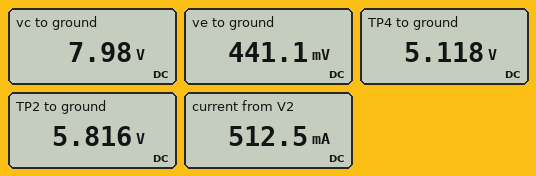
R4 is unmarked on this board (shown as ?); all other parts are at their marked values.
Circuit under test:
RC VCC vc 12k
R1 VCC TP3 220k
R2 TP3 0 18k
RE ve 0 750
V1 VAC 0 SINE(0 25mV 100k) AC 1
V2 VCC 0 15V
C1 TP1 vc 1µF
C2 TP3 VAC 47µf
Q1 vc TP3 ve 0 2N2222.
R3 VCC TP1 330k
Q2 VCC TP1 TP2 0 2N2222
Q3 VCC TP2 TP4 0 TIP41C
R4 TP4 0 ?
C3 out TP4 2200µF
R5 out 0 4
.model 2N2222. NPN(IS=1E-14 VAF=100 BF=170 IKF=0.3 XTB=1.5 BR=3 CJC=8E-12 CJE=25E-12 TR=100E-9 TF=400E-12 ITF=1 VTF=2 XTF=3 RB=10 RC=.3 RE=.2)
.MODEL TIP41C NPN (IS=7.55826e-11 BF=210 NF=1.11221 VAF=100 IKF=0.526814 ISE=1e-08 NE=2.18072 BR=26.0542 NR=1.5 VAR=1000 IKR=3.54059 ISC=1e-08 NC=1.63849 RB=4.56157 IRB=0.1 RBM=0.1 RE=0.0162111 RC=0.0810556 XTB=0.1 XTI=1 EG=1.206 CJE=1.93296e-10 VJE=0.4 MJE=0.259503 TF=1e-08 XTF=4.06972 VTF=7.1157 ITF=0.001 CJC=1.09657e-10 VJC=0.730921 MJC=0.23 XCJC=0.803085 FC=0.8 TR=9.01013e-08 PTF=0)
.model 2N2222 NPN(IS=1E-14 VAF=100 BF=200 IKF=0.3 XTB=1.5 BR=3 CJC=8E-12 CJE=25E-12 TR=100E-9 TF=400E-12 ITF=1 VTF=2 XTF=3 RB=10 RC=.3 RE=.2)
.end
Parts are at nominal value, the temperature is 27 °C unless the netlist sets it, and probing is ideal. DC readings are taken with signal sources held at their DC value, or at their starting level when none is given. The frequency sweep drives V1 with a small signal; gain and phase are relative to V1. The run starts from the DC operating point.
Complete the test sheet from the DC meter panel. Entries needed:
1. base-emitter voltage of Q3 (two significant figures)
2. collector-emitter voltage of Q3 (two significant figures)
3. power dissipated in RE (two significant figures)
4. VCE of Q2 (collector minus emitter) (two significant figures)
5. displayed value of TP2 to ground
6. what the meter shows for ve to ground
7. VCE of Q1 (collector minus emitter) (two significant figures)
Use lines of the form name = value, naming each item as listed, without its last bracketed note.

base-emitter voltage of Q3 = 700 mV
collector-emitter voltage of Q3 = 9.9 V
power dissipated in RE = 260 µW
VCE of Q2 (collector minus emitter) = 9.2 V
displayed value of TP2 to ground = 5.816 V
what the meter shows for ve to ground = 441.1 mV
VCE of Q1 (collector minus emitter) = 7.5 V
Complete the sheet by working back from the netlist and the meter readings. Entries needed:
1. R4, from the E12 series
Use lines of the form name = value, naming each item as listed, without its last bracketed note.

R4, from the E12 series = 10 Ω
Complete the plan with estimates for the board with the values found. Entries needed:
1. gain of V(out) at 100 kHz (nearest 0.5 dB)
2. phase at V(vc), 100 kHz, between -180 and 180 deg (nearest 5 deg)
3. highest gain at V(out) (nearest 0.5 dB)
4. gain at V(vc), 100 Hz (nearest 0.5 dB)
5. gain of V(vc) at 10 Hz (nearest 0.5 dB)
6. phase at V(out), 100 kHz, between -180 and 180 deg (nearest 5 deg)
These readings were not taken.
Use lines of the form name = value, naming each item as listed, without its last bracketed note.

gain of V(out) at 100 kHz = 20.0 dB
phase at V(vc), 100 kHz, between -180 and 180 deg = 165 deg
highest gain at V(out) = 20.5 dB
gain at V(vc), 100 Hz = 21.5 dB
gain of V(vc) at 10 Hz = 22.5 dB
phase at V(out), 100 kHz, between -180 and 180 deg = 160 deg
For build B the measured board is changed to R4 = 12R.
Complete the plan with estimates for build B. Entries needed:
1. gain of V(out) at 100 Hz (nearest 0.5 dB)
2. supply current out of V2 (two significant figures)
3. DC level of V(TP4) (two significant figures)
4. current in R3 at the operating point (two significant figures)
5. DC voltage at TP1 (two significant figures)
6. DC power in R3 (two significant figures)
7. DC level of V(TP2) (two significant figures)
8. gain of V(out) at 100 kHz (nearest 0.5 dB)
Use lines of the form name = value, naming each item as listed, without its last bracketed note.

gain of V(out) at 100 Hz = 20.5 dB
supply current out of V2 = 480 mA
DC level of V(TP4) = 5.7 V
current in R3 at the operating point = 24 µA
DC voltage at TP1 = 7.1 V
DC power in R3 = 190 µW
DC level of V(TP2) = 6.4 V
gain of V(out) at 100 kHz = 20.5 dB
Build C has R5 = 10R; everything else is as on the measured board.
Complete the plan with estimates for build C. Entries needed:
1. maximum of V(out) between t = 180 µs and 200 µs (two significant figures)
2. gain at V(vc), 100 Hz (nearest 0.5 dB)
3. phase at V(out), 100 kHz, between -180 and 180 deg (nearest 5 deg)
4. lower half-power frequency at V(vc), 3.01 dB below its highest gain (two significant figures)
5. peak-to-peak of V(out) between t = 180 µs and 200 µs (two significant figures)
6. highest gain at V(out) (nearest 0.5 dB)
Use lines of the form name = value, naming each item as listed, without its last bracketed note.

maximum of V(out) between t = 180 µs and 200 µs = 290 mV
gain at V(vc), 100 Hz = 22.0 dB
phase at V(out), 100 kHz, between -180 and 180 deg = 165 deg
lower half-power frequency at V(vc), 3.01 dB below its highest gain = 210 mHz
peak-to-peak of V(out) between t = 180 µs and 200 µs = 590 mV
highest gain at V(out) = 21.5 dB
